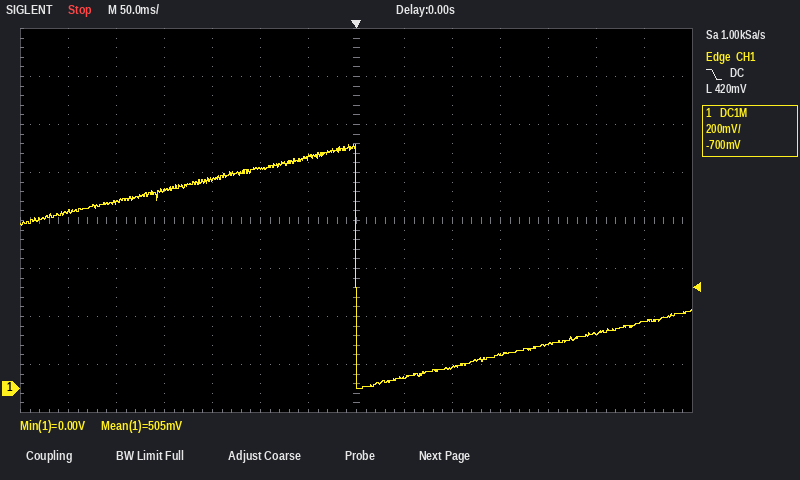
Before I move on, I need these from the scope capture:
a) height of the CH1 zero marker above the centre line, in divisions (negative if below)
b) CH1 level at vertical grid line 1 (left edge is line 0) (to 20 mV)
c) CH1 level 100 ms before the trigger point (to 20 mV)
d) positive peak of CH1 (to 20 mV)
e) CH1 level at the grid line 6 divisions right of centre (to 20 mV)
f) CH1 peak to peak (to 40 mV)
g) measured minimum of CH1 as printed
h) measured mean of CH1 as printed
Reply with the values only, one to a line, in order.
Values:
-3.5 div
740 mV
920 mV
1.02 V
280 mV
1.00 V
0.00 V
505 mV
